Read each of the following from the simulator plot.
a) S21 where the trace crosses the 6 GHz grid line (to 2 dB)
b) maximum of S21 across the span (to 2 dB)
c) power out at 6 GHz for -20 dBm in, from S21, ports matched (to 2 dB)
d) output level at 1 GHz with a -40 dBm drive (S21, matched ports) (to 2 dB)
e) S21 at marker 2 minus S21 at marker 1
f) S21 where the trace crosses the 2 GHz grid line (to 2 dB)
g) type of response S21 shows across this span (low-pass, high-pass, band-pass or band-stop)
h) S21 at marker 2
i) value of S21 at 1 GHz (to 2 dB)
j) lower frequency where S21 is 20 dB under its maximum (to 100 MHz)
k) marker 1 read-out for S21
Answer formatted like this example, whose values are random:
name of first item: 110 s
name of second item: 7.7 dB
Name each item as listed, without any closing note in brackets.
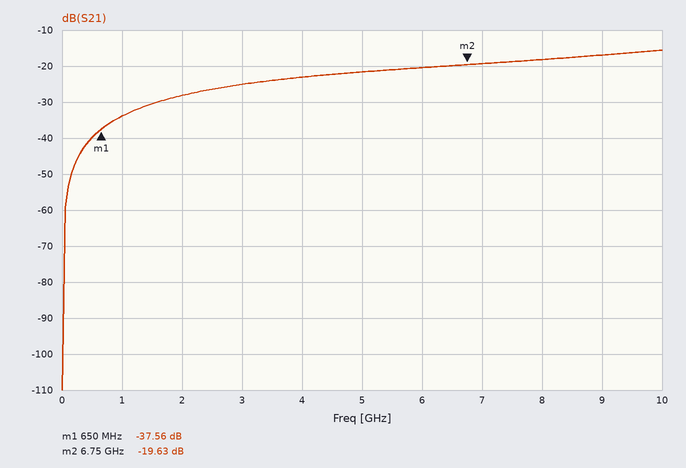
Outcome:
S21 where the trace crosses the 6 GHz grid line: -20 dB
maximum of S21 across the span: -16 dB
power out at 6 GHz for -20 dBm in, from S21, ports matched: -40 dBm
output level at 1 GHz with a -40 dBm drive (S21, matched ports): -74 dBm
S21 at marker 2 minus S21 at marker 1: 17.93 dB
S21 where the trace crosses the 2 GHz grid line: -28 dB
type of response S21 shows across this span: high-pass
S21 at marker 2: -19.63 dB
value of S21 at 1 GHz: -34 dB
lower frequency where S21 is 20 dB under its maximum: 800 MHz
marker 1 read-out for S21: -37.56 dB
